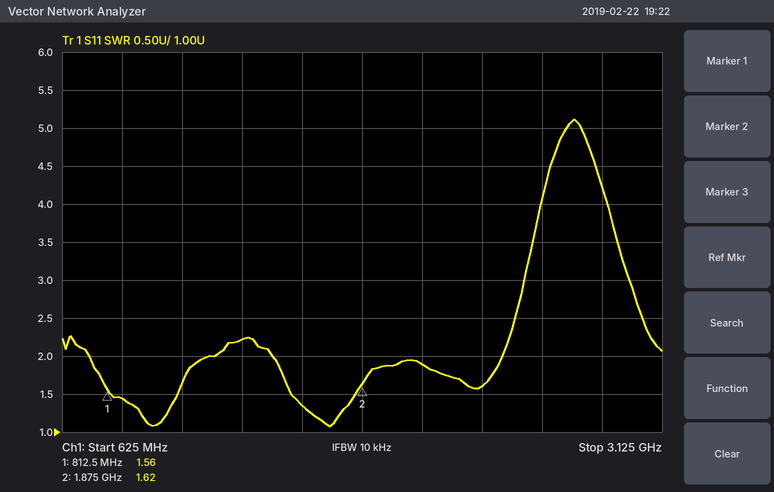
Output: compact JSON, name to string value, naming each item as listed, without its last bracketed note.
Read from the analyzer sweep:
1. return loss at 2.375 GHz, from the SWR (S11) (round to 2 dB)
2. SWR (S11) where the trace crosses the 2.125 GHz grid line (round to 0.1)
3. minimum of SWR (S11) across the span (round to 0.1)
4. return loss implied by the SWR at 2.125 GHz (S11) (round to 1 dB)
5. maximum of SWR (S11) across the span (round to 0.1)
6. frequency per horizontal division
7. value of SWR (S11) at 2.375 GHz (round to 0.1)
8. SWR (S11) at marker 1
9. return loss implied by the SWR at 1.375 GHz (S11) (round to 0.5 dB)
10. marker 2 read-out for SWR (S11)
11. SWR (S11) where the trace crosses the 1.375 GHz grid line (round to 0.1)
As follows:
{"return loss at 2.375 GHz, from the SWR (S11)": "12 dB", "SWR (S11) where the trace crosses the 2.125 GHz grid line": "1.9", "minimum of SWR (S11) across the span": "1.1", "return loss implied by the SWR at 2.125 GHz (S11)": "10 dB", "maximum of SWR (S11) across the span": "5.1", "frequency per horizontal division": "250 MHz", "value of SWR (S11) at 2.375 GHz": "1.6", "SWR (S11) at marker 1": "1.56", "return loss implied by the SWR at 1.375 GHz (S11)": "8.5 dB", "marker 2 read-out for SWR": "1.62", "SWR (S11) where the trace crosses the 1.375 GHz grid line": "2.2"}
